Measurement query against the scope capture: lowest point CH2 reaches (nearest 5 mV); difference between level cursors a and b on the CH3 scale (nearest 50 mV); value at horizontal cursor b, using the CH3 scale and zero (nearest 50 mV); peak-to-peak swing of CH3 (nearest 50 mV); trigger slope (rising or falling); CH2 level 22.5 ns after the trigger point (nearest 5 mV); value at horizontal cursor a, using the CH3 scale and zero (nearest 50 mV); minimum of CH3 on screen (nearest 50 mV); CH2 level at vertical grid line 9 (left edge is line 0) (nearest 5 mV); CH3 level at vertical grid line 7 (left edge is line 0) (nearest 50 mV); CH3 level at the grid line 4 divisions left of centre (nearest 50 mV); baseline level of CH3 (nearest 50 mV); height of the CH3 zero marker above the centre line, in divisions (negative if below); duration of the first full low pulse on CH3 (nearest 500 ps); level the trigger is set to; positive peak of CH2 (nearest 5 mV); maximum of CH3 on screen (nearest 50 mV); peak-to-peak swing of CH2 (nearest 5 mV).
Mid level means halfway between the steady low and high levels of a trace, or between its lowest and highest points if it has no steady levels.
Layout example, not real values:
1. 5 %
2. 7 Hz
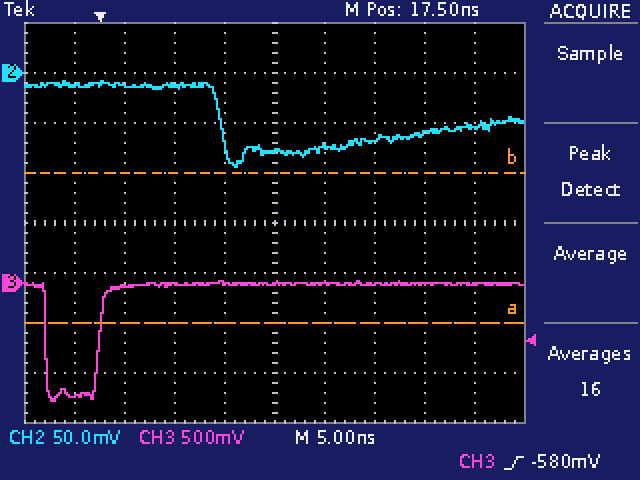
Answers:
1. -95 mV
2. 1.50 V
3. 1.10 V
4. 1.20 V
5. rising
6. -75 mV
7. -400 mV
8. -1.20 V
9. -55 mV
10. 0 mV
11. -1.15 V
12. 0 mV
13. -1.2 div
14. 5.5 ns
15. -580 mV
16. -10 mV
17. 0 mV
18. 85 mV
